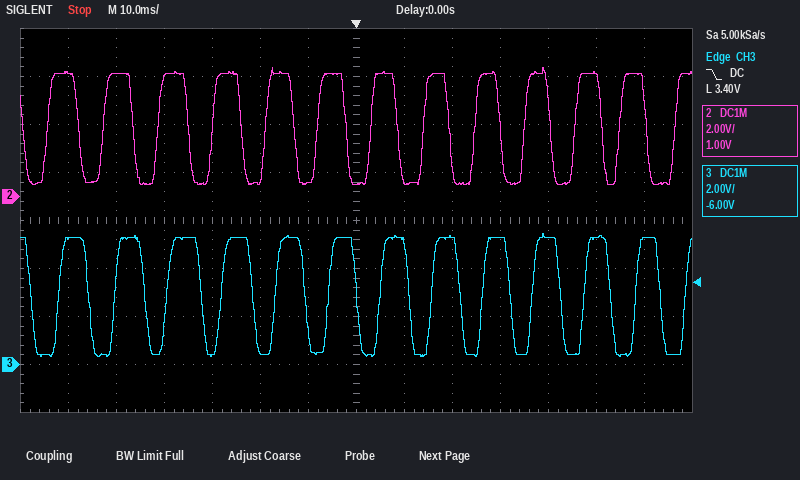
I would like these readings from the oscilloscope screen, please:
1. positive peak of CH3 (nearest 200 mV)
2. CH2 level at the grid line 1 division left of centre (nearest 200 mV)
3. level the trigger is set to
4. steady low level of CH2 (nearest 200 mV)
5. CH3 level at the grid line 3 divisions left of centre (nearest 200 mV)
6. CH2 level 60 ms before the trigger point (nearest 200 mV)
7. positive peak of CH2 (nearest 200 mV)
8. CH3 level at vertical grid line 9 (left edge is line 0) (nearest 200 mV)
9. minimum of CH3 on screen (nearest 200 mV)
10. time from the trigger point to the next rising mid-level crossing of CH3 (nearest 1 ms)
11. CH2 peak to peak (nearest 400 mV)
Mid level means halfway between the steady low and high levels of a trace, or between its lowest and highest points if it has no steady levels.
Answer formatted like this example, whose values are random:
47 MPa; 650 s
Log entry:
5.4 V; 600 mV; 3.40 V; 600 mV; 400 mV; 5.2 V; 5.4 V; 5.4 V; 400 mV; 5 ms; 4.8 V
